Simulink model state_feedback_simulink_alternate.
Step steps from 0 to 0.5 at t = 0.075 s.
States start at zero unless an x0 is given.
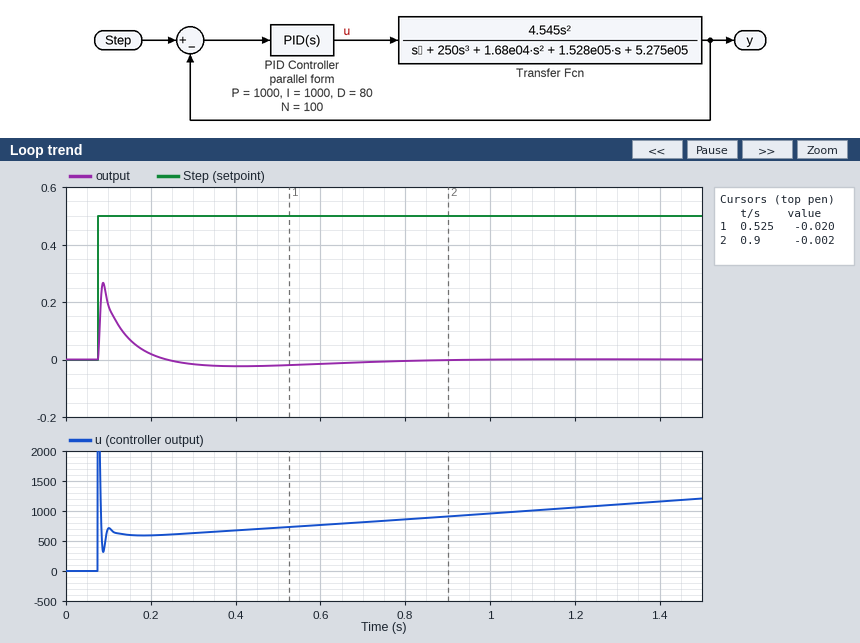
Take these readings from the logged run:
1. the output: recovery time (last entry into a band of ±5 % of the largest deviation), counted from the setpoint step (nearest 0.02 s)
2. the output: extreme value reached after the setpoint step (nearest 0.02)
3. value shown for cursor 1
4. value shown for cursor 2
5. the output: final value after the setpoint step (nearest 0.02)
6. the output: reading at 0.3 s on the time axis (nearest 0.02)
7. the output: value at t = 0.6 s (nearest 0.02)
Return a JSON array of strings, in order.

["0.56 s", "0.26", "-0.020", "-0.002", "0.00", "-0.02", "-0.02"]
